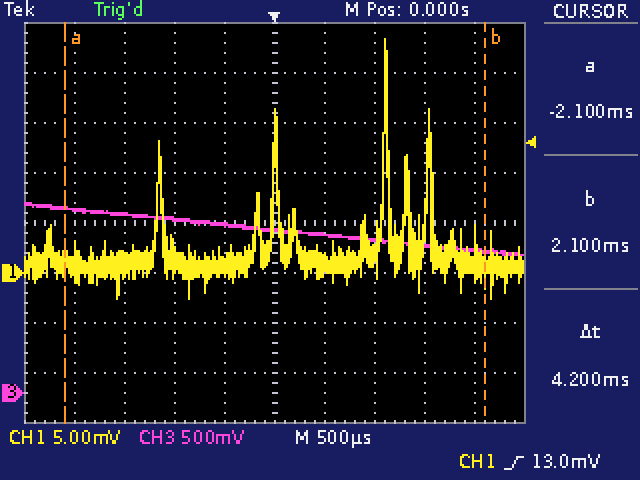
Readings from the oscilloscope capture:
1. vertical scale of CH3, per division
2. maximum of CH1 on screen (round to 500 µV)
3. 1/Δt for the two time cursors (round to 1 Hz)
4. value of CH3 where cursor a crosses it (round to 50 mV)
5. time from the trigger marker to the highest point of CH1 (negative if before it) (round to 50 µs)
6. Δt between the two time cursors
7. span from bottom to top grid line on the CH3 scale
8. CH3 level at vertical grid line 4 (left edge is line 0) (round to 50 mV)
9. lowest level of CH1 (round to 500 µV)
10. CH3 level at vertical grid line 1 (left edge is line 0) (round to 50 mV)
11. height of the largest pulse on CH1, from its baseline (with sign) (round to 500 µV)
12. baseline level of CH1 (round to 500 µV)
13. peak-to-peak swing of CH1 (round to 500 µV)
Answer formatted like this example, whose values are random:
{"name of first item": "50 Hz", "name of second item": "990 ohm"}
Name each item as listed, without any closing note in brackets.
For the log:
{"vertical scale of CH3, per division": "500 mV", "maximum of CH1 on screen": "23.5 mV", "1/Δt for the two time cursors": "238 Hz", "value of CH3 where cursor a crosses it": "1.85 V", "time from the trigger marker to the highest point of CH1 (negative if before it)": "+1.10 ms", "Δt between the two time cursors": "4.2 ms", "span from bottom to top grid line on the CH3 scale": "4 V", "CH3 level at vertical grid line 4 (left edge is line 0)": "1.70 V", "lowest level of CH1": "-2.5 mV", "CH3 level at vertical grid line 1 (left edge is line 0)": "1.85 V", "height of the largest pulse on CH1, from its baseline (with sign)": "+22.5 mV", "baseline level of CH1": "1.0 mV", "peak-to-peak swing of CH1": "26.0 mV"}
